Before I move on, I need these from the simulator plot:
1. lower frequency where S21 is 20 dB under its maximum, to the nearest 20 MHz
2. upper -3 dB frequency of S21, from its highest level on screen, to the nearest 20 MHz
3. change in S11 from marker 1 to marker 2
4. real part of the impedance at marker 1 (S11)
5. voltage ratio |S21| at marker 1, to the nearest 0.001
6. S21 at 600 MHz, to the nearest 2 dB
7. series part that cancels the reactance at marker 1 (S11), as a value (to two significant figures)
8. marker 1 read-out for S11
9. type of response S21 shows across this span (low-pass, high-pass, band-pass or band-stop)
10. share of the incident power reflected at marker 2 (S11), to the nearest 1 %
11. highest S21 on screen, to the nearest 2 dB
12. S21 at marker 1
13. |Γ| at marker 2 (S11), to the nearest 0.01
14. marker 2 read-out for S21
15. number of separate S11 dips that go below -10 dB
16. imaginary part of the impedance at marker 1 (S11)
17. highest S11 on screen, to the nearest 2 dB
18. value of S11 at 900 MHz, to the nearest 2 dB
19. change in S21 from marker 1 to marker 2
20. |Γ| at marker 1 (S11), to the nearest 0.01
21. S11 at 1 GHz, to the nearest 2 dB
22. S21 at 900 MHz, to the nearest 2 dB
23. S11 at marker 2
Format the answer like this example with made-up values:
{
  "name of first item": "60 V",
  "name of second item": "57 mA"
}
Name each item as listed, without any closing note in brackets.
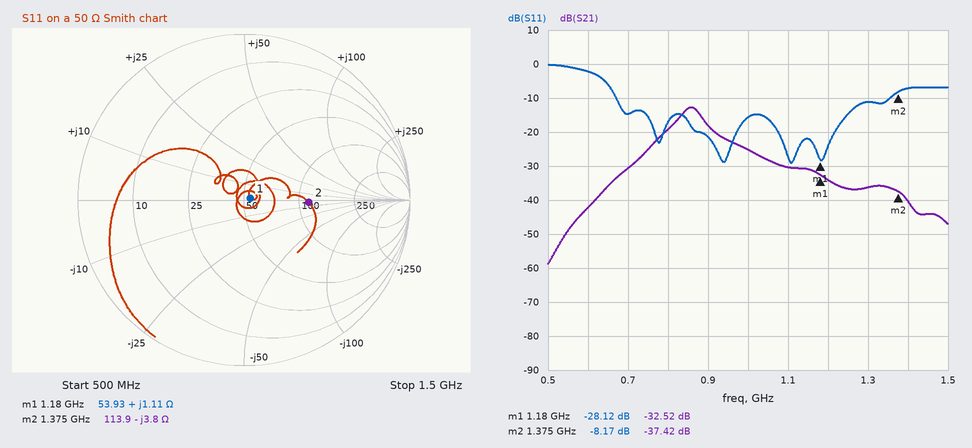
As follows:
{
  "lower frequency where S21 is 20 dB under its maximum, to the nearest 20 MHz": "680 MHz",
  "upper -3 dB frequency of S21, from its highest level on screen, to the nearest 20 MHz": "880 MHz",
  "change in S11 from marker 1 to marker 2": "19.95 dB",
  "real part of the impedance at marker 1": "53.93 Ω",
  "voltage ratio |S21| at marker 1, to the nearest 0.001": "0.024",
  "S21 at 600 MHz, to the nearest 2 dB": "-42 dB",
  "series part that cancels the reactance at marker 1 (S11), as a value": "120 pF",
  "marker 1 read-out for S11": "-28.12 dB",
  "type of response S21 shows across this span": "band-pass",
  "share of the incident power reflected at marker 2 (S11), to the nearest 1 %": "15 %",
  "highest S21 on screen, to the nearest 2 dB": "-12 dB",
  "S21 at marker 1": "-32.52 dB",
  "|Γ| at marker 2 (S11), to the nearest 0.01": "0.39",
  "marker 2 read-out for S21": "-37.42 dB",
  "number of separate S11 dips that go below -10 dB": "4",
  "imaginary part of the impedance at marker 1": "+1.11 Ω",
  "highest S11 on screen, to the nearest 2 dB": "0 dB",
  "value of S11 at 900 MHz, to the nearest 2 dB": "-22 dB",
  "change in S21 from marker 1 to marker 2": "-4.90 dB",
  "|Γ| at marker 1 (S11), to the nearest 0.01": "0.04",
  "S11 at 1 GHz, to the nearest 2 dB": "-16 dB",
  "S21 at 900 MHz, to the nearest 2 dB": "-18 dB",
  "S11 at marker 2": "-8.17 dB"
}
